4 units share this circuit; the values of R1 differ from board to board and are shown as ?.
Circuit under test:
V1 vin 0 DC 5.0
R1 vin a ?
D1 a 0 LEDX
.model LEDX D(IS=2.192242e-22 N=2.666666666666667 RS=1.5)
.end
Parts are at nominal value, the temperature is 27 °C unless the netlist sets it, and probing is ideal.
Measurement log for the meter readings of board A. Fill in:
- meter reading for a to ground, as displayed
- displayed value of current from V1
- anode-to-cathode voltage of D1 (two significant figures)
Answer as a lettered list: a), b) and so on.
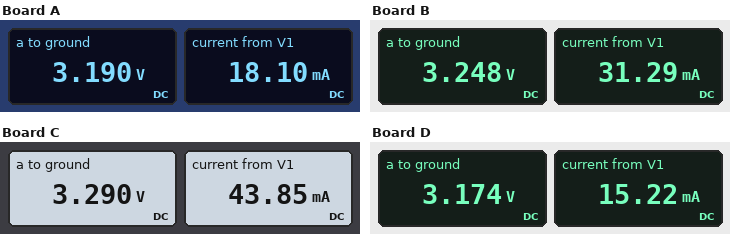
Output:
a) 3.190 V
b) 18.10 mA
c) 3.2 V
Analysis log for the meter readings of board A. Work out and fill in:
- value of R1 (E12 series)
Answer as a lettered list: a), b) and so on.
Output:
a) 100 Ω
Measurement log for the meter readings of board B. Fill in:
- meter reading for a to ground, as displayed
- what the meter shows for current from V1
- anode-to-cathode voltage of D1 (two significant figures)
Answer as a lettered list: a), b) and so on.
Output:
a) 3.248 V
b) 31.29 mA
c) 3.2 V
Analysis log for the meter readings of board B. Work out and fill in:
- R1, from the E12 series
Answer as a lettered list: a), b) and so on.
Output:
a) 56 Ω
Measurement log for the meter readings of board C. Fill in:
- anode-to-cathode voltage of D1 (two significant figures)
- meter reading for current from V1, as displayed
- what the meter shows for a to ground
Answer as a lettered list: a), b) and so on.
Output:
a) 3.3 V
b) 43.85 mA
c) 3.290 V
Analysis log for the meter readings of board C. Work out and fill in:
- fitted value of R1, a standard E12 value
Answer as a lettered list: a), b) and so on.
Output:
a) 39 Ω
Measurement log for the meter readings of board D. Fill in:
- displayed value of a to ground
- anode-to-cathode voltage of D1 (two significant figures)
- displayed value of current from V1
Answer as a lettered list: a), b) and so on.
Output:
a) 3.174 V
b) 3.2 V
c) 15.22 mA
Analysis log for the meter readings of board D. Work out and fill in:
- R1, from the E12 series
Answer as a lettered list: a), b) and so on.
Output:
a) 120 Ω
